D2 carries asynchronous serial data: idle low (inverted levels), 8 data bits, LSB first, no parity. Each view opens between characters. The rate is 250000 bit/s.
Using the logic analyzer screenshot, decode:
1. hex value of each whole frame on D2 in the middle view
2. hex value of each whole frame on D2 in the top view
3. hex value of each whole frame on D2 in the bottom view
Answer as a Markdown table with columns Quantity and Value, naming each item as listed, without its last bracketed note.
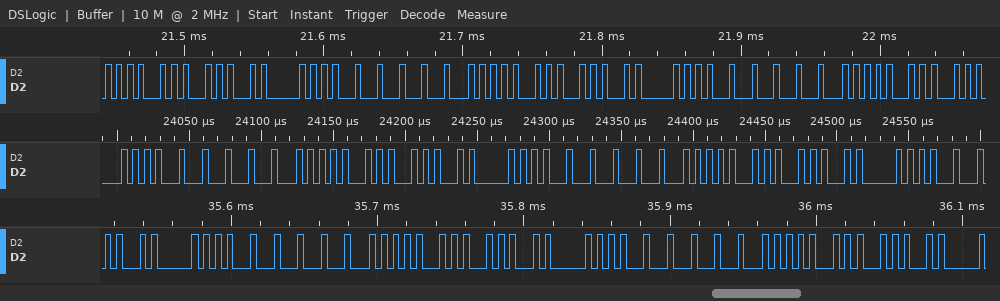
| Quantity | Value |
|---|---|
| hex value of each whole frame on D2 in the middle view | D5, 77, 77, D5, 75, 5D, D5, 77, 77, D5, 75, 5D, D5 |
| hex value of each whole frame on D2 in the top view | D5, 75, 5D, D5, 77, 77, D5, 75, 5D, D5, 77, 77, D5, 75 |
| hex value of each whole frame on D2 in the bottom view | 5D, D5, 77, 77, D5, 75, 5D, D5, 77, 77, D5, 75, 5D |
